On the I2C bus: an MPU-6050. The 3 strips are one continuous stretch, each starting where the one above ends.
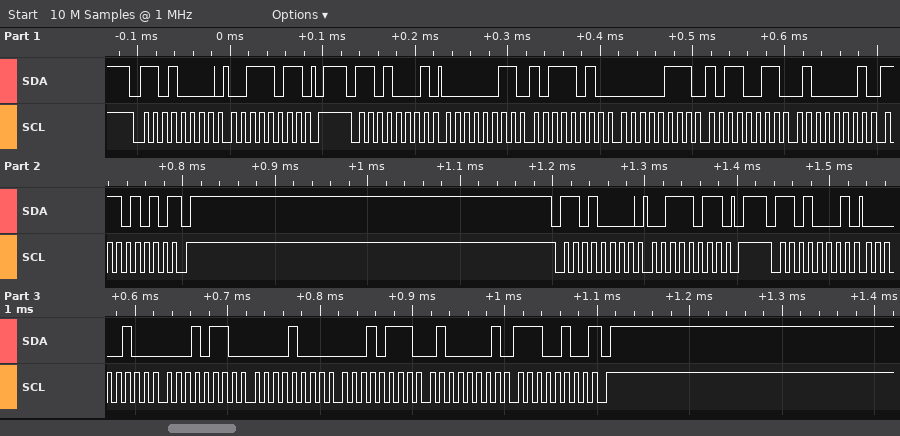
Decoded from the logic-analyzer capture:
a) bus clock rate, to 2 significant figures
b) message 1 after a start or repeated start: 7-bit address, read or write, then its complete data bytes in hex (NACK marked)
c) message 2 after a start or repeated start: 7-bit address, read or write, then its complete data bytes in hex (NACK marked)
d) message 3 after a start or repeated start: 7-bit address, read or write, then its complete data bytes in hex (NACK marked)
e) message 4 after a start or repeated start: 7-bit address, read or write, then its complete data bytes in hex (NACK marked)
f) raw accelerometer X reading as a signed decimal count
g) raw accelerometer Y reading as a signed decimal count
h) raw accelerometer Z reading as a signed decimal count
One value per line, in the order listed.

100 kHz
0x68 write: 3B
0x68 read: 03 BA 07 B3 41 EA NACK
0x68 write: 3B
0x68 read: 04 16 08 17 41 E4 NACK
954
1971
16874
